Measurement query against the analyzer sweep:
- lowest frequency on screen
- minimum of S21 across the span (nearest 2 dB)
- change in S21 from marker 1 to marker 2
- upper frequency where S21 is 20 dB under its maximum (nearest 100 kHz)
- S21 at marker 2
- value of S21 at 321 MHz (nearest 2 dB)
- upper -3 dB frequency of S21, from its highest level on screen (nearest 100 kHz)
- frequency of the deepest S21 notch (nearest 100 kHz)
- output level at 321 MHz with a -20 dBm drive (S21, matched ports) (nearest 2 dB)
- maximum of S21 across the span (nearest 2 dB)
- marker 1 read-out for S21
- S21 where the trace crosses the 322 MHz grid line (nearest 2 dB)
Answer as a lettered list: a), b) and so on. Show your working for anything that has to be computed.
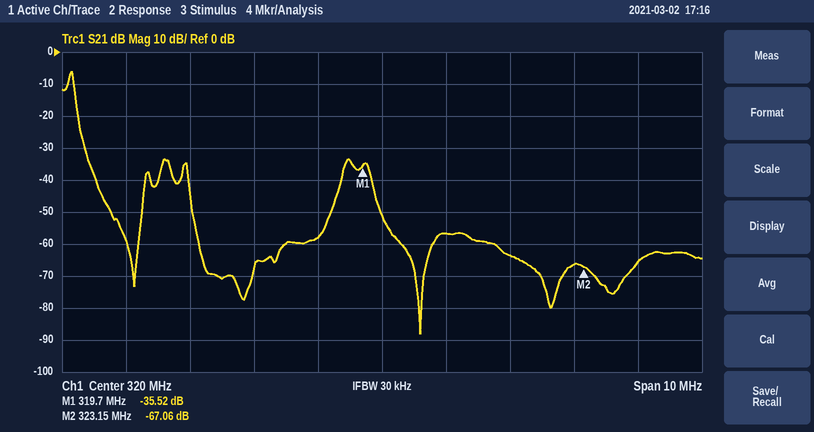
a) 315 MHz
b) -88 dB
c) -67.06 − (-35.52) = -31.54 dB
d) 315.3 MHz
e) -67.06 dB
f) -56 dB
g) 315.2 MHz
h) 320.6 MHz
i) -20 dBm + (-56 dB) = -76 dBm
j) -6 dB
k) -35.52 dB
l) -64 dB
